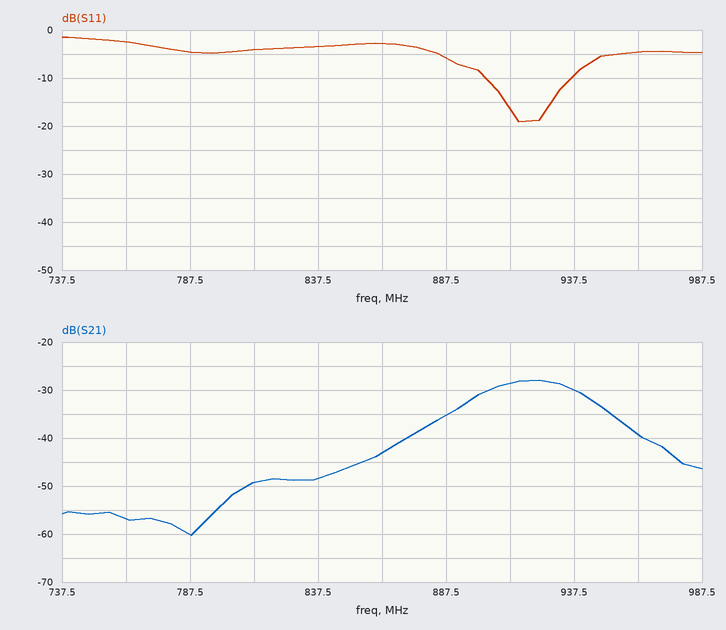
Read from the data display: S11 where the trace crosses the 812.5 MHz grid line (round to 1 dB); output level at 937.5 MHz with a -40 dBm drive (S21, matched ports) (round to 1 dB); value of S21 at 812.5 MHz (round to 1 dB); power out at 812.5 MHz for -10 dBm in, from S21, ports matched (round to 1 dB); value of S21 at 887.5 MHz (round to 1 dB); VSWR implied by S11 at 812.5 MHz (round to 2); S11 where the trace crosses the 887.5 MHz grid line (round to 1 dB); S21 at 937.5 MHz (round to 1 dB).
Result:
-4 dB
-70 dBm
-49 dB
-59 dBm
-35 dB
4
-6 dB
-30 dB
